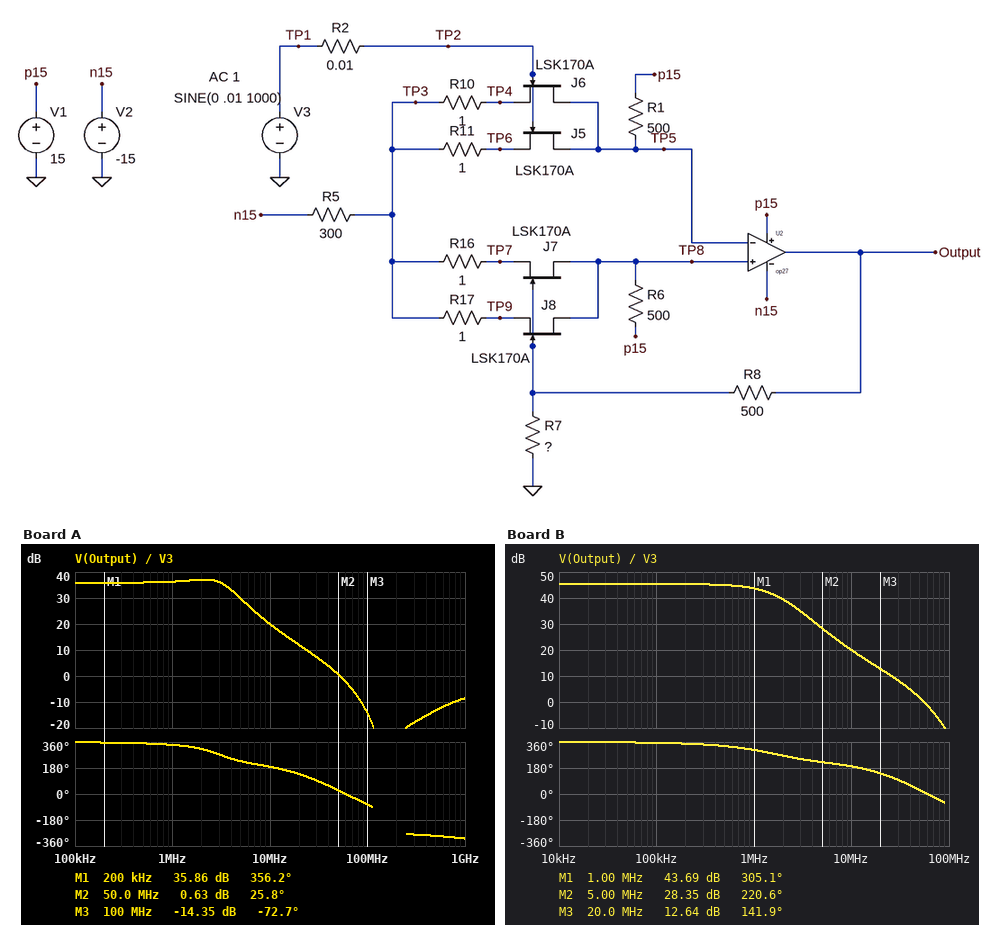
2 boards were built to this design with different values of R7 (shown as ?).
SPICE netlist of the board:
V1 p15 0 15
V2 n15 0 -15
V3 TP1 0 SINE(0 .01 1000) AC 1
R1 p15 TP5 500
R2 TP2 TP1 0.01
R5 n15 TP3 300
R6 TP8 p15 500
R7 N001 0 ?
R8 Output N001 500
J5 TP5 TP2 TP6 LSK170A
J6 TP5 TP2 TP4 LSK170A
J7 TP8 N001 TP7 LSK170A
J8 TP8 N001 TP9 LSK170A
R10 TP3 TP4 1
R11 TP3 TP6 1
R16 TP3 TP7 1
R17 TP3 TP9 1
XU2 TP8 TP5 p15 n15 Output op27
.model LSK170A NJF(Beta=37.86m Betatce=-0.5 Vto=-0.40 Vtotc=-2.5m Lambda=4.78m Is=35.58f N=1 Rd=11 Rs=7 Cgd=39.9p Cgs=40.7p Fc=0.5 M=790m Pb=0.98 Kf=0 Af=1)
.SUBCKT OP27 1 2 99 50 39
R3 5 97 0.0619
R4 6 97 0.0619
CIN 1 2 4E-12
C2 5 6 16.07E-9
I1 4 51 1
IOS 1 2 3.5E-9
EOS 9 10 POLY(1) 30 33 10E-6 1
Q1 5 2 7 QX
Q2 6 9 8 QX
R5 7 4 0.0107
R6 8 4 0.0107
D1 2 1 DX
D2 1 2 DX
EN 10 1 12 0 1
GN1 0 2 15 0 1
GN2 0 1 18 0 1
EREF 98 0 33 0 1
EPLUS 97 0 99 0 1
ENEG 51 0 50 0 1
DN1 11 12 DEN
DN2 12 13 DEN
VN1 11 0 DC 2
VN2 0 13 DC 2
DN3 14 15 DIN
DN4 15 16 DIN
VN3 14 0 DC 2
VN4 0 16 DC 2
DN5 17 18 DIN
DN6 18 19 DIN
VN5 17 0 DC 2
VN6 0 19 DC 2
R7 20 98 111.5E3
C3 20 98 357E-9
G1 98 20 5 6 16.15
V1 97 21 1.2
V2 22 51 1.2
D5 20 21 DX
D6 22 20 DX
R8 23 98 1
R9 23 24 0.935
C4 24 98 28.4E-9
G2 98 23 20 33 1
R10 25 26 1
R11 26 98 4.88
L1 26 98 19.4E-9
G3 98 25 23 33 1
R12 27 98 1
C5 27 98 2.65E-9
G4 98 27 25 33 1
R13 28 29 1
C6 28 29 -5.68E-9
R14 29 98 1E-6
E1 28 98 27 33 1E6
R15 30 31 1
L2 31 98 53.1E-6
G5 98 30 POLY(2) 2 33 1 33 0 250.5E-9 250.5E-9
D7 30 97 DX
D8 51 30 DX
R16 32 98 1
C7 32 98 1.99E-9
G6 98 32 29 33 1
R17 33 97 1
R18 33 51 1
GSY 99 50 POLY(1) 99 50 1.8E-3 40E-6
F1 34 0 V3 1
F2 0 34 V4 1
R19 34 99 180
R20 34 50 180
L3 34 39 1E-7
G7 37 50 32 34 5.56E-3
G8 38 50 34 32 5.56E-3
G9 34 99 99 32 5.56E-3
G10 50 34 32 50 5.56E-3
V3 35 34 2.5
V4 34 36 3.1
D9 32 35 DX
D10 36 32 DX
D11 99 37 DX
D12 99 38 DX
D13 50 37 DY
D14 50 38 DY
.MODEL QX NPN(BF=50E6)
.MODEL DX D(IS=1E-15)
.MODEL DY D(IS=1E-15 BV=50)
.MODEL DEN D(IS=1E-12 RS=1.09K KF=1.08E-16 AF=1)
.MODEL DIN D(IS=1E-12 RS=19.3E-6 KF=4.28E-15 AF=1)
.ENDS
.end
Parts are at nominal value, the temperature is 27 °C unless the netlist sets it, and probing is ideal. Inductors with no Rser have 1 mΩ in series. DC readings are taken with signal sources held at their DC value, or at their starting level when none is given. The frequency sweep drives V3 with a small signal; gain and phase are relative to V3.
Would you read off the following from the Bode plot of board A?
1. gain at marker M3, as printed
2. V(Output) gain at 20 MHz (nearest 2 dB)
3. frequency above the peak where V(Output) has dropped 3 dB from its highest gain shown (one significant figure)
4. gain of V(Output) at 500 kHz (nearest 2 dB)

-14.35 dB
12 dB
4 MHz
36 dB
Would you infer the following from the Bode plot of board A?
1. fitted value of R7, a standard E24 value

8.2 Ω
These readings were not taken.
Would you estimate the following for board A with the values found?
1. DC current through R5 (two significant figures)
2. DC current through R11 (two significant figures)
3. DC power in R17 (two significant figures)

49 mA
12 mA
150 µW
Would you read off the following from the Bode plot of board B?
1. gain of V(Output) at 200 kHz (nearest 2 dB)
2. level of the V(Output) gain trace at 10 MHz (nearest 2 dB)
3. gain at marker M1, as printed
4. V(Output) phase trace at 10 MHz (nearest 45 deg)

46 dB
20 dB
43.69 dB
180 deg
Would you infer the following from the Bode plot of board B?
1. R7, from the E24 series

2.7 Ω
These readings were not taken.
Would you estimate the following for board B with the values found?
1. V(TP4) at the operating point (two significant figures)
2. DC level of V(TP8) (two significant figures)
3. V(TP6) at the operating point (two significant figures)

-250 mV
2.7 V
-250 mV
